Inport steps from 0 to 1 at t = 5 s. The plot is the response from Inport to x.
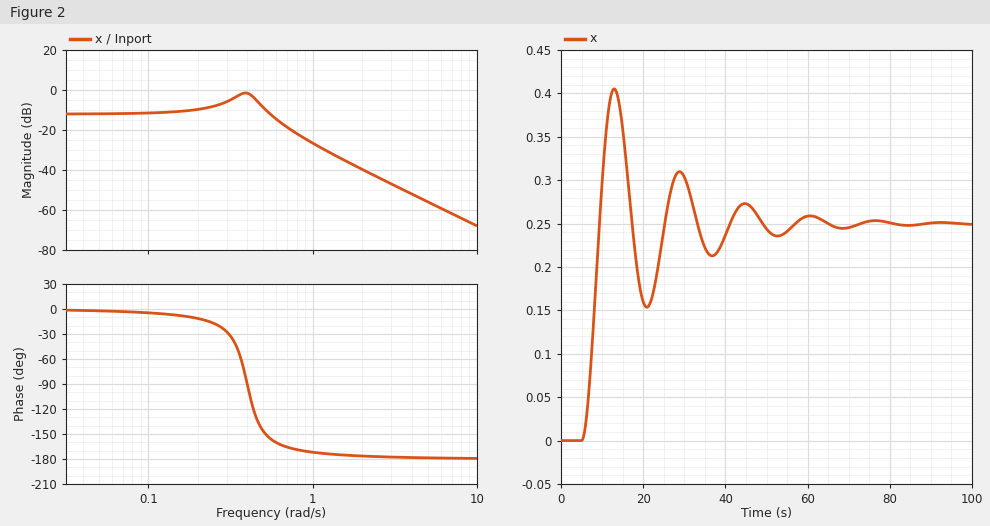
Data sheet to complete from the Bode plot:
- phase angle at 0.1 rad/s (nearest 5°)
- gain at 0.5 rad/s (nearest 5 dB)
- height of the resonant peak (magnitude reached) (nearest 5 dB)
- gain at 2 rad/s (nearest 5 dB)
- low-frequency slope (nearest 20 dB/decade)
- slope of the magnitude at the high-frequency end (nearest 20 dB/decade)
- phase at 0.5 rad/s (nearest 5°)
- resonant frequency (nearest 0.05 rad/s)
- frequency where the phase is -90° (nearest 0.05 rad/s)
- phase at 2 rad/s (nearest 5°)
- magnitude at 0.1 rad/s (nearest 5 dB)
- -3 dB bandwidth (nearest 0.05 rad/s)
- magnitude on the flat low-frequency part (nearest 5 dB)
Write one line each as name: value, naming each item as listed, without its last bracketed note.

phase angle at 0.1 rad/s: -5°
gain at 0.5 rad/s: -10 dB
height of the resonant peak (magnitude reached): 0 dB
gain at 2 rad/s: -40 dB
low-frequency slope: 0 dB/decade
slope of the magnitude at the high-frequency end: -40 dB/decade
phase at 0.5 rad/s: -145°
resonant frequency: 0.40 rad/s
frequency where the phase is -90°: 0.40 rad/s
phase at 2 rad/s: -175°
magnitude at 0.1 rad/s: -10 dB
-3 dB bandwidth: 0.60 rad/s
magnitude on the flat low-frequency part: -10 dB
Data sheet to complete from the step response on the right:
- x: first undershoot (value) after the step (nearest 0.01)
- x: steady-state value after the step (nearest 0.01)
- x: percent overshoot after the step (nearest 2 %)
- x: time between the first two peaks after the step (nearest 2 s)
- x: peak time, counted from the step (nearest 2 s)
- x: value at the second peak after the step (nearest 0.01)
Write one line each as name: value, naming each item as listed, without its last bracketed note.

x: first undershoot (value) after the step: 0.15
x: steady-state value after the step: 0.25
x: percent overshoot after the step: 62 %
x: time between the first two peaks after the step: 16 s
x: peak time, counted from the step: 8 s
x: value at the second peak after the step: 0.31
